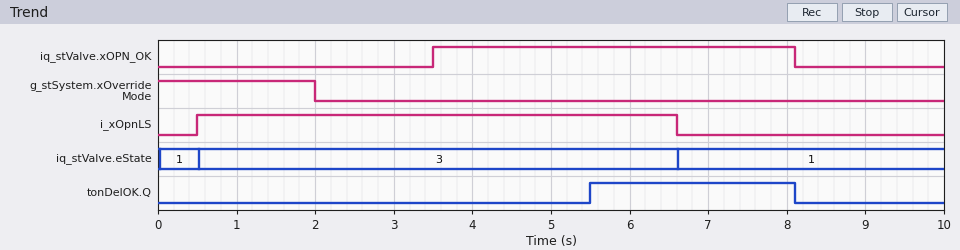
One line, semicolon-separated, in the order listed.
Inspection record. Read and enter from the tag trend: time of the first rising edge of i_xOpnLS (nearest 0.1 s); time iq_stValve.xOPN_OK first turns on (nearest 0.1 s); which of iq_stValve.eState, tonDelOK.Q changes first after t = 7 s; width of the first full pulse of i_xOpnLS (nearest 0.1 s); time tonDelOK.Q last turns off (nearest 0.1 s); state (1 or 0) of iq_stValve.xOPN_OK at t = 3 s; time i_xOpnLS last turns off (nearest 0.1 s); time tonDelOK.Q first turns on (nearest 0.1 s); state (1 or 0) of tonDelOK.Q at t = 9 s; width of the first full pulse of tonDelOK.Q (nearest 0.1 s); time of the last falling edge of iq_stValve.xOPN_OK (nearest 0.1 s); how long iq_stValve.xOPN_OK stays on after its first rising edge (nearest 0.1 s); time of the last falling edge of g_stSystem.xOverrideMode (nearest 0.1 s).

0.5 s; 3.5 s; tonDelOK.Q; 6.1 s; 8.1 s; 0; 6.6 s; 5.5 s; 0; 2.6 s; 8.1 s; 4.6 s; 2.0 s
